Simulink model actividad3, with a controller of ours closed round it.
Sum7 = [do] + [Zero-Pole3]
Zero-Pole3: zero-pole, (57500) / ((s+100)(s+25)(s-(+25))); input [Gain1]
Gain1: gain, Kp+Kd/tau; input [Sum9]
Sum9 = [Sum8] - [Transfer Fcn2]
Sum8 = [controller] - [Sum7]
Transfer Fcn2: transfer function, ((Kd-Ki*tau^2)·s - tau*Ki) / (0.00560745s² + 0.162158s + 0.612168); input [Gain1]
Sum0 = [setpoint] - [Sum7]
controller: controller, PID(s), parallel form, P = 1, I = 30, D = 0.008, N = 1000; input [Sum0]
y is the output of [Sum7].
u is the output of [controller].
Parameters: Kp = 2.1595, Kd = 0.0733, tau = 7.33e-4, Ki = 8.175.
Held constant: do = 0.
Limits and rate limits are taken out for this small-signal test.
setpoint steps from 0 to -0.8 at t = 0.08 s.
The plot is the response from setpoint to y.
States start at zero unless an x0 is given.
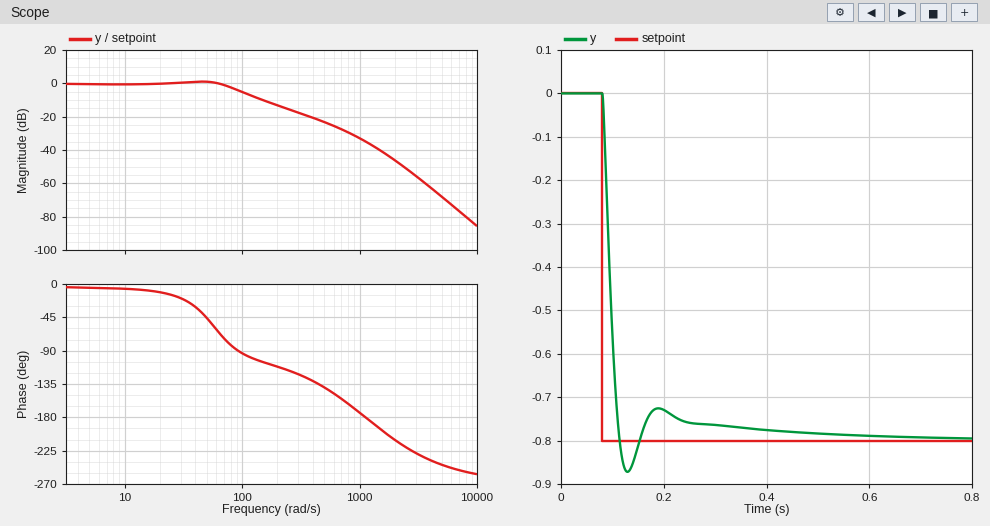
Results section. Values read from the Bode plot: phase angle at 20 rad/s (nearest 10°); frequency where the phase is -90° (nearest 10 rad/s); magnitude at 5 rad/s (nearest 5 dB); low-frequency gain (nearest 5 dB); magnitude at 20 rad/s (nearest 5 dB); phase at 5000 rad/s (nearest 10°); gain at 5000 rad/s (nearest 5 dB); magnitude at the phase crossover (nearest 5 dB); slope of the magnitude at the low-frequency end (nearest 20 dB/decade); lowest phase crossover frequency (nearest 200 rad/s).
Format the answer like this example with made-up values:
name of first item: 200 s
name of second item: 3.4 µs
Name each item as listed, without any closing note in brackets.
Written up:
phase angle at 20 rad/s: -10°
frequency where the phase is -90°: 90 rad/s
magnitude at 5 rad/s: 0 dB
low-frequency gain: 0 dB
magnitude at 20 rad/s: 0 dB
phase at 5000 rad/s: -240°
gain at 5000 rad/s: -70 dB
magnitude at the phase crossover: -35 dB
slope of the magnitude at the low-frequency end: 0 dB/decade
lowest phase crossover frequency: 1200 rad/s
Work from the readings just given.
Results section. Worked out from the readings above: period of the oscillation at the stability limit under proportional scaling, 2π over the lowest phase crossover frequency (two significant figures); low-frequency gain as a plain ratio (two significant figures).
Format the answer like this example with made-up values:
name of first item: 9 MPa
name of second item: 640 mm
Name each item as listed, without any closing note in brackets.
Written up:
period of the oscillation at the stability limit under proportional scaling, 2π over the lowest phase crossover frequency: 0.0052 s
low-frequency gain as a plain ratio: 1.0
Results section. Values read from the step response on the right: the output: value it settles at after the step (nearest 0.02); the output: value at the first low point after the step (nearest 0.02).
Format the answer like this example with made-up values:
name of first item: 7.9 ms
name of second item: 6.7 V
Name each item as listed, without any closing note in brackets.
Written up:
the output: value it settles at after the step: -0.80
the output: value at the first low point after the step: -0.88
